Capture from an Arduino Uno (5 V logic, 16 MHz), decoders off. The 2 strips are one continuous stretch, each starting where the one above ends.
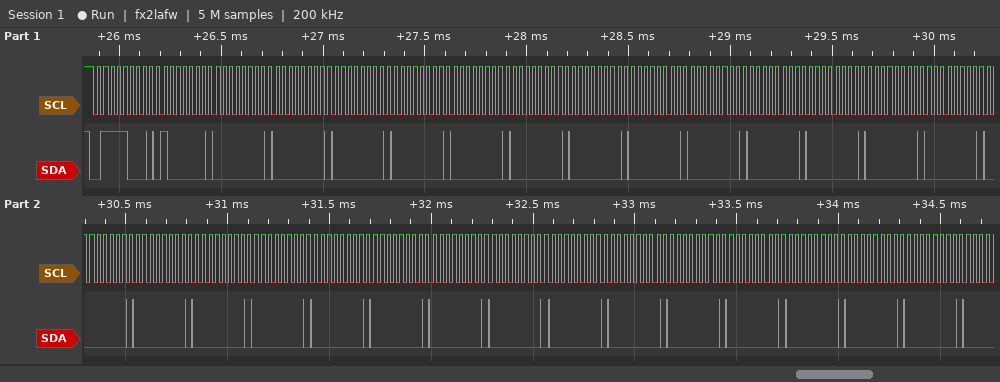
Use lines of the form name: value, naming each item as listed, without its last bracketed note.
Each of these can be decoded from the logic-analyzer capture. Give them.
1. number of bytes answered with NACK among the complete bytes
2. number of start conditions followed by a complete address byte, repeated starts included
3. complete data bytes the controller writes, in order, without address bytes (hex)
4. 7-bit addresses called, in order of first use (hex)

number of bytes answered with NACK among the complete bytes: 0
number of start conditions followed by a complete address byte, repeated starts included: 1
complete data bytes the controller writes, in order, without address bytes: 40 00 00 00 00 00 00 00 00 00 00 00 00 00 00 00 00 00 00 00 00 00 00 00 00 00 00 00 00
7-bit addresses called, in order of first use: 0x3C
